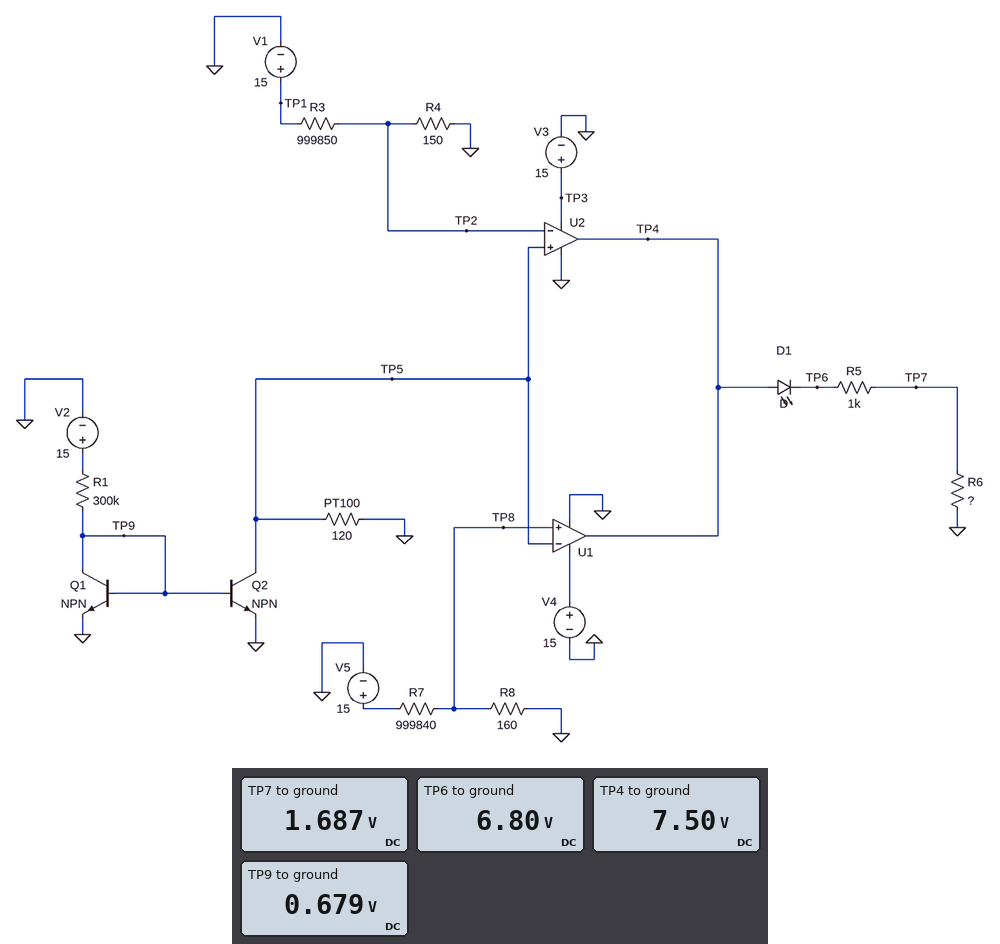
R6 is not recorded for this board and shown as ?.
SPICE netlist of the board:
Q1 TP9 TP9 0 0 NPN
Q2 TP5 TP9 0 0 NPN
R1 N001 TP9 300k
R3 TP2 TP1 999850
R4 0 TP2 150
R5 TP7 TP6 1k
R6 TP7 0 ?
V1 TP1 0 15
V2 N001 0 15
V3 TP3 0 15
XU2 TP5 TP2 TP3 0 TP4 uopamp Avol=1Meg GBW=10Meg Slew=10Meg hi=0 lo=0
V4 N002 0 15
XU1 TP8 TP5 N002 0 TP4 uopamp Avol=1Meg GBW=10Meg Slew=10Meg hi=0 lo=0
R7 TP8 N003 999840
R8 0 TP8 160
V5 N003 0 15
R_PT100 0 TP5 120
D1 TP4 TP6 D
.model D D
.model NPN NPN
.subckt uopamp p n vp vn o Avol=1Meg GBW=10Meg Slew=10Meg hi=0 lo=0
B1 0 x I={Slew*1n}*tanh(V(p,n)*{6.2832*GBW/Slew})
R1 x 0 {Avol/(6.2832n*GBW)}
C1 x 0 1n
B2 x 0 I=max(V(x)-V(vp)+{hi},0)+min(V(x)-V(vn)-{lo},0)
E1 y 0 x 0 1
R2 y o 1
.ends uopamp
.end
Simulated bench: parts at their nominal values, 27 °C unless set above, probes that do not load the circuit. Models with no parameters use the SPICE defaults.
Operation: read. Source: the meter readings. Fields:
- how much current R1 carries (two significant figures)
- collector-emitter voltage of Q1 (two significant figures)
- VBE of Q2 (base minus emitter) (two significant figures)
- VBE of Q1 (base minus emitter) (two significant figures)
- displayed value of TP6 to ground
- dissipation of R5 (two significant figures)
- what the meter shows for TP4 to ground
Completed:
48 µA
680 mV
680 mV
680 mV
6.80 V
26 mW
7.50 V
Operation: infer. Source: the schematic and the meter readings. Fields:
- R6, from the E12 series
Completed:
330 Ω
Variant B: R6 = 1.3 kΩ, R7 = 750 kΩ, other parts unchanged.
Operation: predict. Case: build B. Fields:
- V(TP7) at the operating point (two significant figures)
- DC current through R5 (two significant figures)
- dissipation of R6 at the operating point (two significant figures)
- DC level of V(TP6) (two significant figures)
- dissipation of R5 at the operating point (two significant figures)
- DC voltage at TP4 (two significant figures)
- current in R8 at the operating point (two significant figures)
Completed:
8.1 V
6.2 mA
50 mW
14 V
39 mW
15 V
20 µA
